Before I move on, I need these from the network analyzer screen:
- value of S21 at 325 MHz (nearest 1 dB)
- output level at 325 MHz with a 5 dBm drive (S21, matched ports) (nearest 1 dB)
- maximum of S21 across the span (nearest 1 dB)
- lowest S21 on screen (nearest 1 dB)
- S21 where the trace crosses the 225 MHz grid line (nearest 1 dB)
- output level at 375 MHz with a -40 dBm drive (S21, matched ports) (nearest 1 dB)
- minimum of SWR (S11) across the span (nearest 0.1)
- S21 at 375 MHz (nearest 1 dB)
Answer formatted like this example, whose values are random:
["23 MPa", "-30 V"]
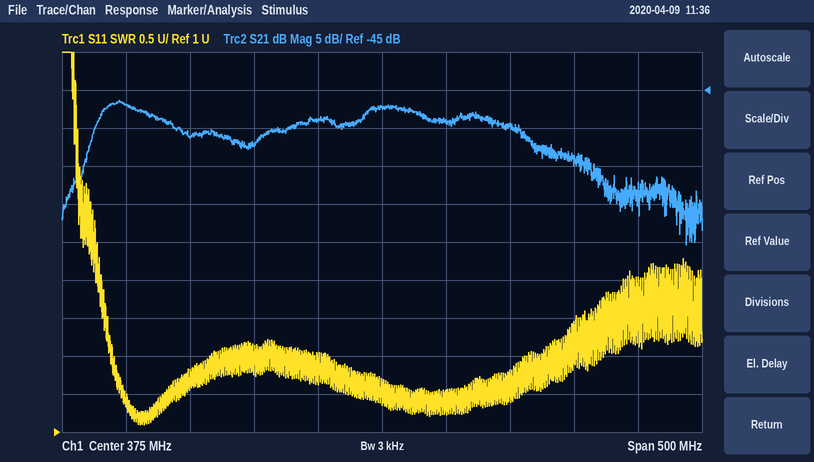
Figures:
["-49 dB", "-44 dBm", "-46 dB", "-65 dB", "-51 dB", "-87 dBm", "1.1", "-47 dB"]
